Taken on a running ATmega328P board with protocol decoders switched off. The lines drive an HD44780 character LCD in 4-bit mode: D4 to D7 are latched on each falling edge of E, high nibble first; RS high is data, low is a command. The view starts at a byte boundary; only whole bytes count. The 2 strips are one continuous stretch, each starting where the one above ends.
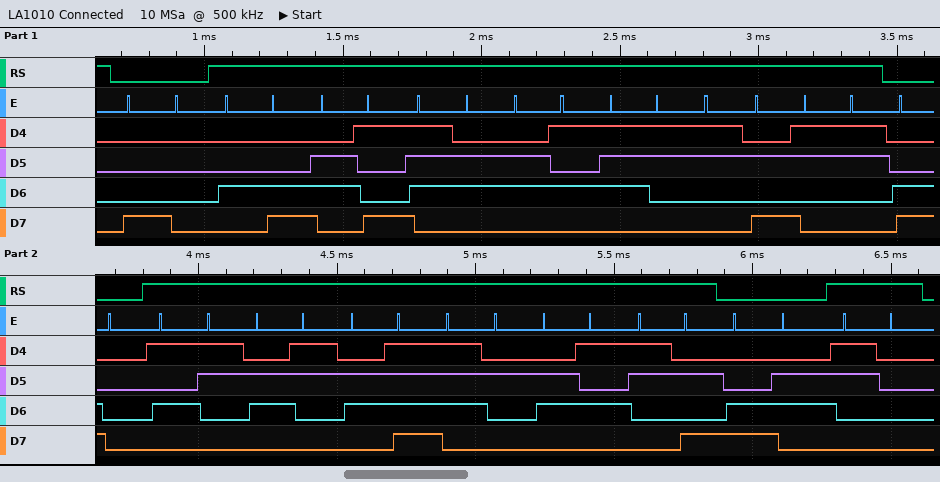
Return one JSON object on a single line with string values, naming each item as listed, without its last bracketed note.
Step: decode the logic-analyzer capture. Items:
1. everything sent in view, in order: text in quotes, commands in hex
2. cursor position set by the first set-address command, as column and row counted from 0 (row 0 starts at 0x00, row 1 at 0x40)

{"everything sent in view, in order: text in quotes, commands in hex": "0x80 \"Lives:3\" 0xC0 \"Score:\" 0xC6 \"0\"", "cursor position set by the first set-address command, as column and row counted from 0": "column 0, row 0"}
